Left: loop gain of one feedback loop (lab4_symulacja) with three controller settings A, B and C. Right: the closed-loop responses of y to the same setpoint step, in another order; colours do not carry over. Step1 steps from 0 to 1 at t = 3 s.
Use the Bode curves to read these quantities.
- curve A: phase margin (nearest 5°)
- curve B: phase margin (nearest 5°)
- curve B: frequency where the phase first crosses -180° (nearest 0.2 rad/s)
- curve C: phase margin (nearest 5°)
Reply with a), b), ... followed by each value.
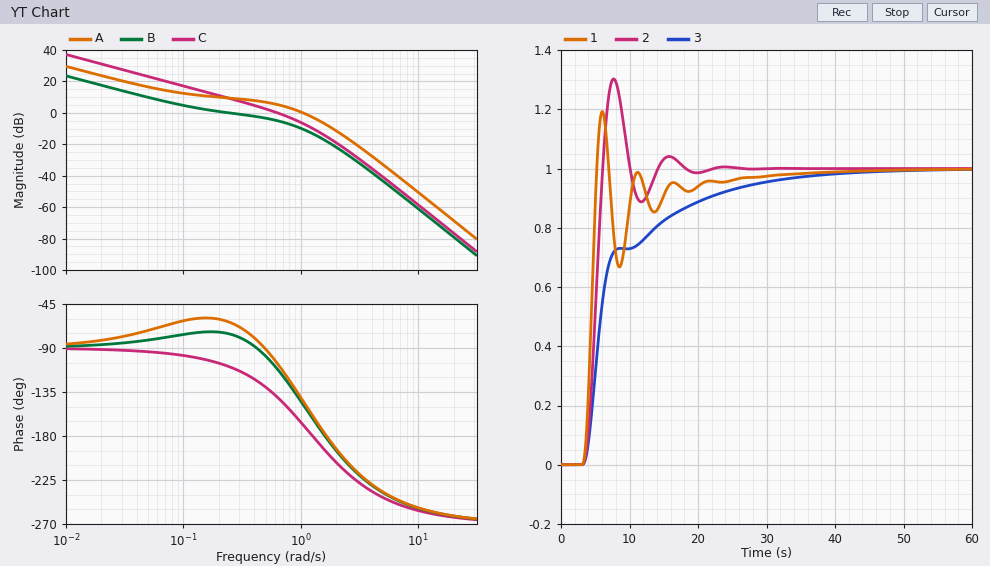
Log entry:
a) 35°
b) 105°
c) 1.6 rad/s
d) 40°
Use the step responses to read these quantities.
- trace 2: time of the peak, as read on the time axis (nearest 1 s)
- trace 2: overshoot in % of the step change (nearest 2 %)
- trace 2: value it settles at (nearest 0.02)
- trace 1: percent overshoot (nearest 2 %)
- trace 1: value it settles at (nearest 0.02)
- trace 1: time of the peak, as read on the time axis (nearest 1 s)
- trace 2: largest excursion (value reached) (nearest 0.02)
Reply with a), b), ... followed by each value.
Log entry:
a) 8 s
b) 30 %
c) 1.00
d) 20 %
e) 1.00
f) 6 s
g) 1.30
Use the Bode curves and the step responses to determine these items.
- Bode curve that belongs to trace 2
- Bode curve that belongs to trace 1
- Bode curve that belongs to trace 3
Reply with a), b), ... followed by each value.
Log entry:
a) C
b) A
c) B
